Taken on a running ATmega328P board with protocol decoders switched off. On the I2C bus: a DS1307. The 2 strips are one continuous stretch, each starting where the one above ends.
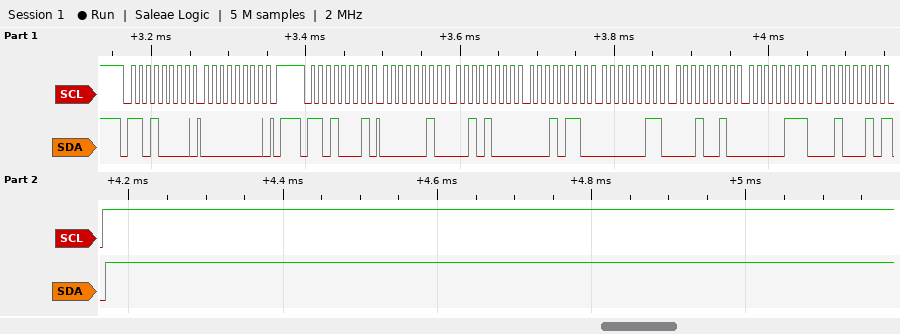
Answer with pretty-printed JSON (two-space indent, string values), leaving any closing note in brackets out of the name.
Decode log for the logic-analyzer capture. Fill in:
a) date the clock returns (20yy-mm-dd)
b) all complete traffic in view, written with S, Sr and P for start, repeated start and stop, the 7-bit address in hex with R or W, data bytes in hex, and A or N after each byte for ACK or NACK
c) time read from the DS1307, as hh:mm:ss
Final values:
{
  "date the clock returns": "2022-07-12",
  "all complete traffic in view, written with S, Sr and P for start, repeated start and stop, the 7-bit address in hex with R or W, data bytes in hex, and A or N after each byte for ACK or NACK": "S 68W A 00 A P S 68R A 02 A 28 A 16 A 03 A 12 A 07 A 22 N P",
  "time read from the DS1307, as hh:mm:ss": "16:28:02"
}
